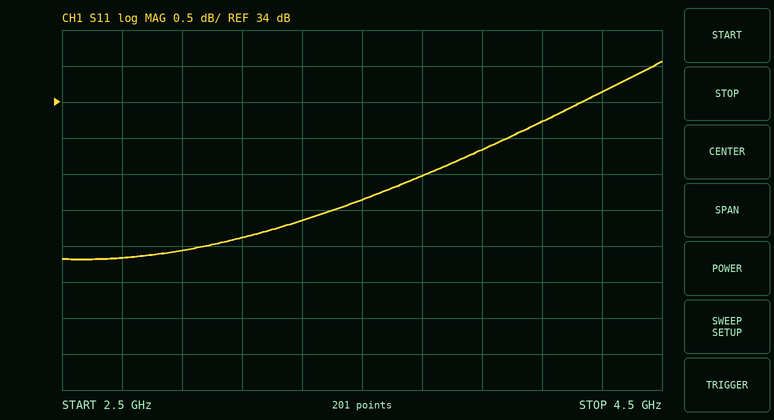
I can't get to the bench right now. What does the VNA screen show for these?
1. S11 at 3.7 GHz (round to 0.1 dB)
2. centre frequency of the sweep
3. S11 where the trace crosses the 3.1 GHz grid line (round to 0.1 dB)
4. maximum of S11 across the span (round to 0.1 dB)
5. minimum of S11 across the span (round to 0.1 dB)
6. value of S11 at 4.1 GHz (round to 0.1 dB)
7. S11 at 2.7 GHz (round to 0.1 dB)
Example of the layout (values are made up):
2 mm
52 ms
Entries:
33.0 dB
3.5 GHz
32.1 dB
34.6 dB
31.8 dB
33.7 dB
31.8 dB
